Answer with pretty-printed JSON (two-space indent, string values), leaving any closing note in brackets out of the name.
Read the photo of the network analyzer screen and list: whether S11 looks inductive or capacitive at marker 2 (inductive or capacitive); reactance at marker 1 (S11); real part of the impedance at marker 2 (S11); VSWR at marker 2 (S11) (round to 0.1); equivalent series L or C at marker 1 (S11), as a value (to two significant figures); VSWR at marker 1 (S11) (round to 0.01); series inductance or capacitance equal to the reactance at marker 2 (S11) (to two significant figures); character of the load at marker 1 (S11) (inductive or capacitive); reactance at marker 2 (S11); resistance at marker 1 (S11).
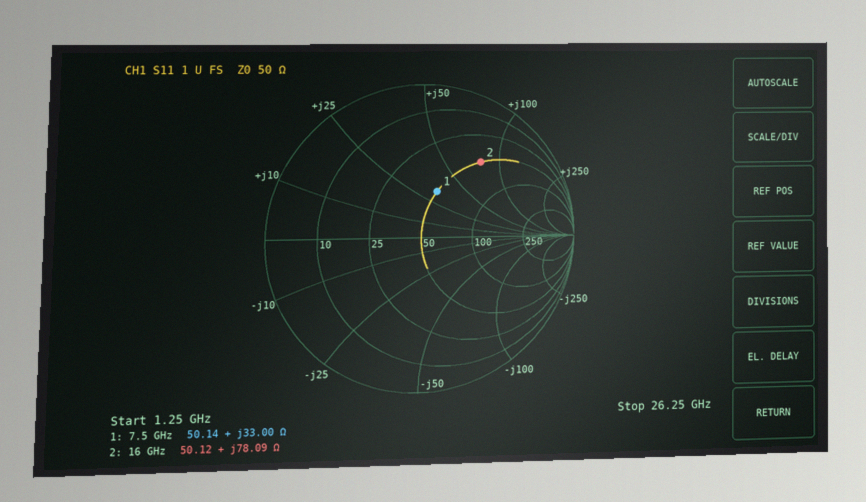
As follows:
{
  "whether S11 looks inductive or capacitive at marker 2": "inductive",
  "reactance at marker 1": "+33.00 Ω",
  "real part of the impedance at marker 2": "50.12 Ω",
  "VSWR at marker 2 (S11)": "4.2",
  "equivalent series L or C at marker 1 (S11), as a value": "700 pH",
  "VSWR at marker 1 (S11)": "1.91",
  "series inductance or capacitance equal to the reactance at marker 2 (S11)": "780 pH",
  "character of the load at marker 1 (S11)": "inductive",
  "reactance at marker 2": "+78.09 Ω",
  "resistance at marker 1": "50.14 Ω"
}
